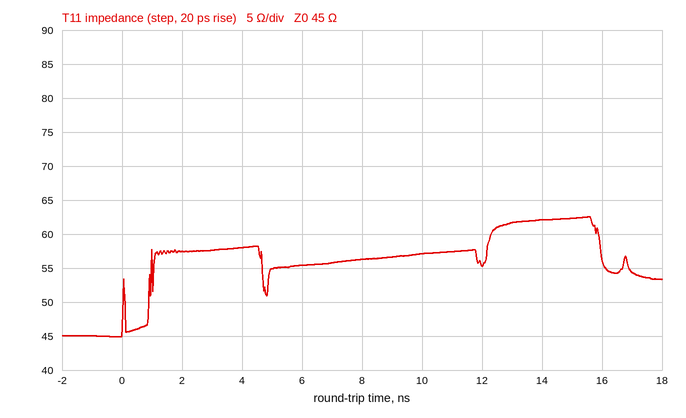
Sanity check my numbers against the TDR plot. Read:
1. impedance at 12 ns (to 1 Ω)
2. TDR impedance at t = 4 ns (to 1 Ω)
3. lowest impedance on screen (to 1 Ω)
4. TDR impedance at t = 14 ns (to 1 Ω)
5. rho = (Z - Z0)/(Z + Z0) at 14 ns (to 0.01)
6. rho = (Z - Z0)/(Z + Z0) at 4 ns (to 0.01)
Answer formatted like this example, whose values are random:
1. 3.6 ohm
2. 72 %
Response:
1. 55 Ω
2. 58 Ω
3. 45 Ω
4. 62 Ω
5. +0.16
6. +0.13
